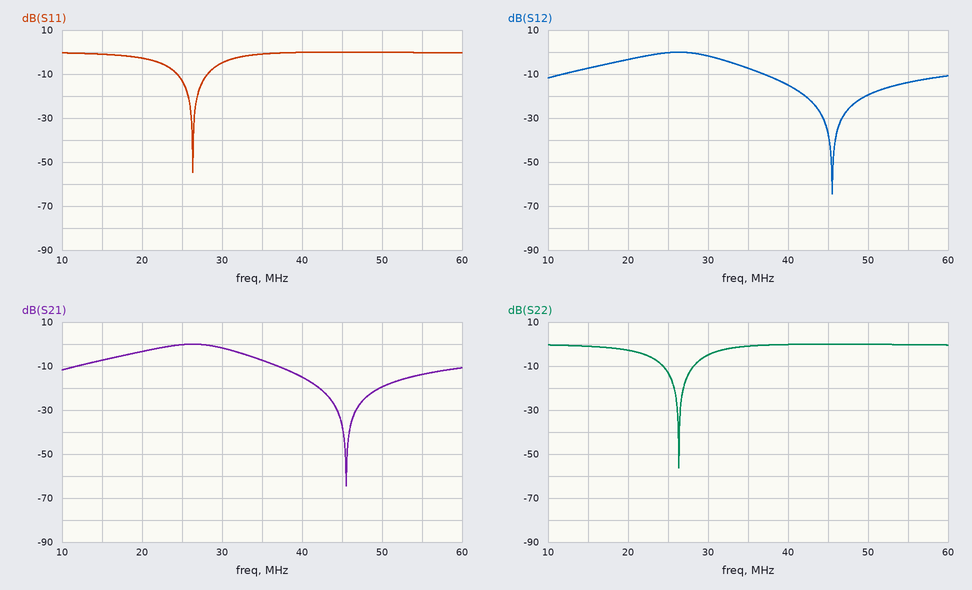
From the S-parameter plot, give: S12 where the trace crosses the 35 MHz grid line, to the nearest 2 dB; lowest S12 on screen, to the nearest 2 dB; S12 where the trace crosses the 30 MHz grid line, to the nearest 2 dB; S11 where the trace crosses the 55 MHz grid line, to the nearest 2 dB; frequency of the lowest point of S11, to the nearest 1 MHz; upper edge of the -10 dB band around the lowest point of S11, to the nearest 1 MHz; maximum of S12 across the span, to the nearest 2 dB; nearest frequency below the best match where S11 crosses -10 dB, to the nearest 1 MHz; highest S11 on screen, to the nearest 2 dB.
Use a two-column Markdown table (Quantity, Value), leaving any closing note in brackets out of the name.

| Quantity | Value |
|---|---|
| S12 where the trace crosses the 35 MHz grid line, to the nearest 2 dB | -8 dB |
| lowest S12 on screen, to the nearest 2 dB | -64 dB |
| S12 where the trace crosses the 30 MHz grid line, to the nearest 2 dB | -2 dB |
| S11 where the trace crosses the 55 MHz grid line, to the nearest 2 dB | 0 dB |
| frequency of the lowest point of S11, to the nearest 1 MHz | 26 MHz |
| upper edge of the -10 dB band around the lowest point of S11, to the nearest 1 MHz | 28 MHz |
| maximum of S12 across the span, to the nearest 2 dB | 0 dB |
| nearest frequency below the best match where S11 crosses -10 dB, to the nearest 1 MHz | 24 MHz |
| highest S11 on screen, to the nearest 2 dB | 0 dB |
